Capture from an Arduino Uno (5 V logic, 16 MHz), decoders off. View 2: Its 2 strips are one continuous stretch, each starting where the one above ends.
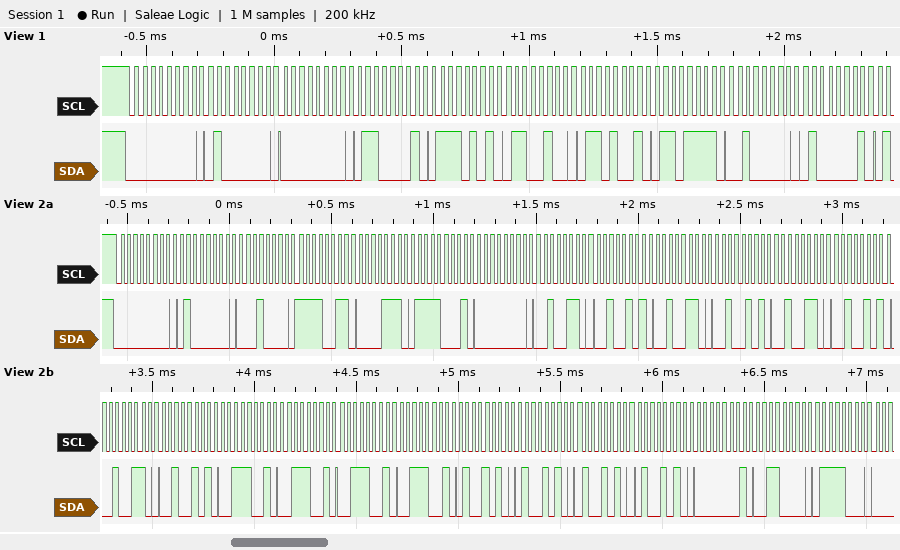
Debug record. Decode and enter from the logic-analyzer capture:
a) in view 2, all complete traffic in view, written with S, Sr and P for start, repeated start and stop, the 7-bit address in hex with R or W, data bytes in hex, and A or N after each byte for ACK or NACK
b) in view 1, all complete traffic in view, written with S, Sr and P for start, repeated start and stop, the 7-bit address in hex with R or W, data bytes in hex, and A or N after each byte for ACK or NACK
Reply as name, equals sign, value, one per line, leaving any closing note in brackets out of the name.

in view 2, all complete traffic in view, written with S, Sr and P for start, repeated start and stop, the 7-bit address in hex with R or W, data bytes in hex, and A or N after each byte for ACK or NACK = S 00W A 40 A 10 A F3 A 0E A F1 A 00 A 26 A 25 A 26 A 25 A 26 A 25 A 26 A 25 A 39 A 39 A 39 A 39 A 4A A 4A A 4A A 4A A 01 A 30 A 78 A
in view 1, all complete traffic in view, written with S, Sr and P for start, repeated start and stop, the 7-bit address in hex with R or W, data bytes in hex, and A or N after each byte for ACK or NACK = S 00W A 40 A 00 A 61 A 75 A 64 A 69 A 6F A 20 A 41 A
